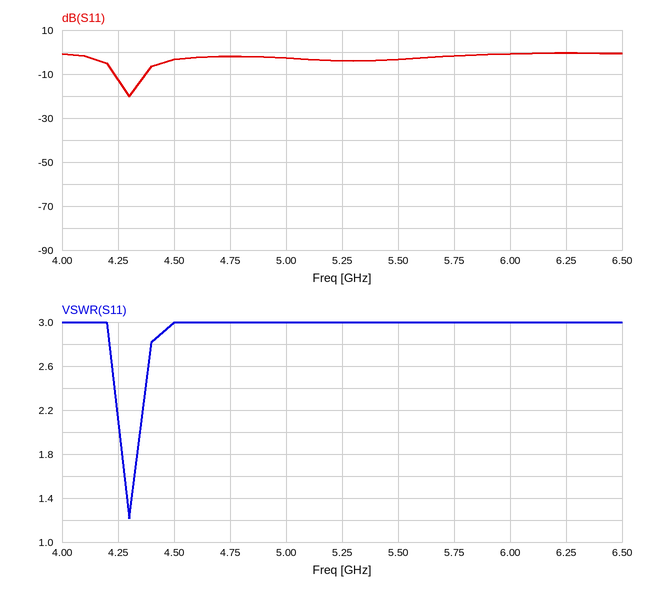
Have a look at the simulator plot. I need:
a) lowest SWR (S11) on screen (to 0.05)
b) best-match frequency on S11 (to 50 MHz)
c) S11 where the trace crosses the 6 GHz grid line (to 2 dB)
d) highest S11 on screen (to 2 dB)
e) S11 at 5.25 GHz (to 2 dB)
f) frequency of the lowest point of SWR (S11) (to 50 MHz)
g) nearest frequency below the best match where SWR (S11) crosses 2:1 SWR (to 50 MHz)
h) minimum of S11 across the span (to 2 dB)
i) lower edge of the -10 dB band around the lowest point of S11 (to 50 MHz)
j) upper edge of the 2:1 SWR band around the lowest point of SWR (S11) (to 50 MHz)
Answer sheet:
1.20
4.30 GHz
0 dB
0 dB
-4 dB
4.30 GHz
4.25 GHz
-20 dB
4.25 GHz
4.35 GHz
